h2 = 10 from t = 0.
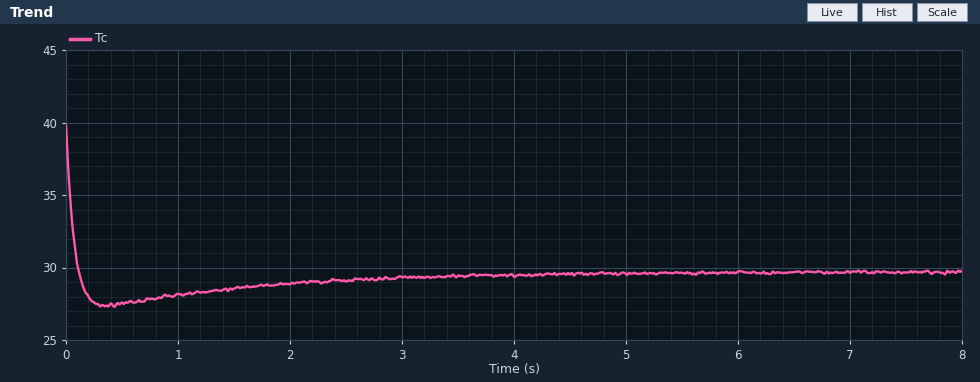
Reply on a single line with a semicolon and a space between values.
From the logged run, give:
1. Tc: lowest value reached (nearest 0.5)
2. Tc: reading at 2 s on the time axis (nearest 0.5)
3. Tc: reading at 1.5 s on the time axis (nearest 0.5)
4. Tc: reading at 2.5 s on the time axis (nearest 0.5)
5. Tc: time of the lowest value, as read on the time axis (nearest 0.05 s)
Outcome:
27.5; 29.0; 28.5; 29.0; 0.35 s
